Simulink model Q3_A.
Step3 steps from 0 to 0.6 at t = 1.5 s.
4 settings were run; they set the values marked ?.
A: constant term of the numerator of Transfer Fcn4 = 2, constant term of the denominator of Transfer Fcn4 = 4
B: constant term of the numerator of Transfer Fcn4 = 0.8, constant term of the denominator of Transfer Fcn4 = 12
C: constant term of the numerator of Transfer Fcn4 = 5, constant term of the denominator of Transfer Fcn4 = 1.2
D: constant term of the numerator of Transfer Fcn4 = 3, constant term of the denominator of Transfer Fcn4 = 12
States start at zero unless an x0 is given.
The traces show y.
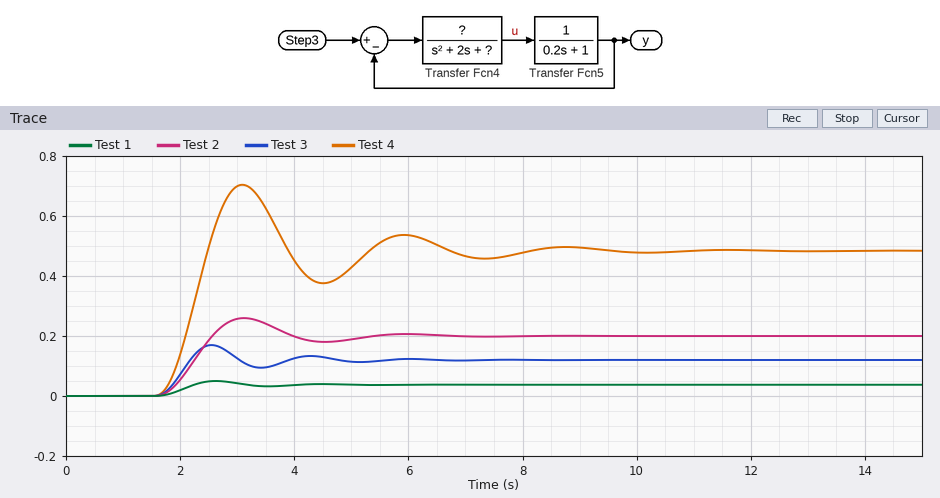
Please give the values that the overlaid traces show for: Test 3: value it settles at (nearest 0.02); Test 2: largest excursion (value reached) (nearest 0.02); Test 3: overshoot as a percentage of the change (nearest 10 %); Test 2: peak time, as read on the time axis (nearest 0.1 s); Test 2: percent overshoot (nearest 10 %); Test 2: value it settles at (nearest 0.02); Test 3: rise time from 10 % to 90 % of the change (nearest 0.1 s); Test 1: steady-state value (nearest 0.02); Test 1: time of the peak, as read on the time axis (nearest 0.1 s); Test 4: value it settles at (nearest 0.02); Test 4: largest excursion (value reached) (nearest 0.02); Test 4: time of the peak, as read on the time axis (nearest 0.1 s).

0.12
0.26
40 %
3.1 s
30 %
0.20
0.4 s
0.04
2.6 s
0.48
0.70
3.1 s
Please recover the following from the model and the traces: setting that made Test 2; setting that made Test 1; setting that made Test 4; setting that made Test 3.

A
B
C
D
